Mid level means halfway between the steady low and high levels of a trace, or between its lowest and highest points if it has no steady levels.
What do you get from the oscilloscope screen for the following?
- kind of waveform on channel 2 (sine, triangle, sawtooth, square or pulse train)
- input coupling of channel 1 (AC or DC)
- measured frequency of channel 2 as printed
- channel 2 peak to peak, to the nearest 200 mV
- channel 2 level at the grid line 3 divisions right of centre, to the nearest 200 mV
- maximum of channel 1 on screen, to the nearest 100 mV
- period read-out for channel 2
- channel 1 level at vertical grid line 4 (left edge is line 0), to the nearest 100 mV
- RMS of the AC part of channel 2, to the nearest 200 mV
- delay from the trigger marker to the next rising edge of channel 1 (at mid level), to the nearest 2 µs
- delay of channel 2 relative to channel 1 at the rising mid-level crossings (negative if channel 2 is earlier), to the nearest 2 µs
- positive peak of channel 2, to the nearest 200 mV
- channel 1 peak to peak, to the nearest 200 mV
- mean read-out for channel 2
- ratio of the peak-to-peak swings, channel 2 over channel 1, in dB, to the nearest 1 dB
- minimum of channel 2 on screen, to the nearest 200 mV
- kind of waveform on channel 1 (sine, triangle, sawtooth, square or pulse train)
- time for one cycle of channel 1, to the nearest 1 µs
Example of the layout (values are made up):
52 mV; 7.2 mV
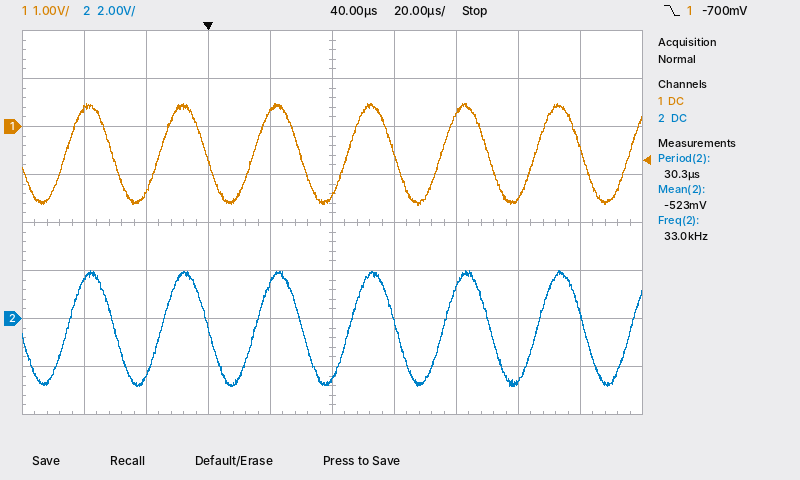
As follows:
sine; DC; 33.0 kHz; 4.8 V; -2.6 V; 500 mV; 30.3 µs; 300 mV; 1.6 V; 14 µs; 0 µs; 2.0 V; 2.2 V; -523 mV; 7 dB; -2.8 V; sine; 30 µs
